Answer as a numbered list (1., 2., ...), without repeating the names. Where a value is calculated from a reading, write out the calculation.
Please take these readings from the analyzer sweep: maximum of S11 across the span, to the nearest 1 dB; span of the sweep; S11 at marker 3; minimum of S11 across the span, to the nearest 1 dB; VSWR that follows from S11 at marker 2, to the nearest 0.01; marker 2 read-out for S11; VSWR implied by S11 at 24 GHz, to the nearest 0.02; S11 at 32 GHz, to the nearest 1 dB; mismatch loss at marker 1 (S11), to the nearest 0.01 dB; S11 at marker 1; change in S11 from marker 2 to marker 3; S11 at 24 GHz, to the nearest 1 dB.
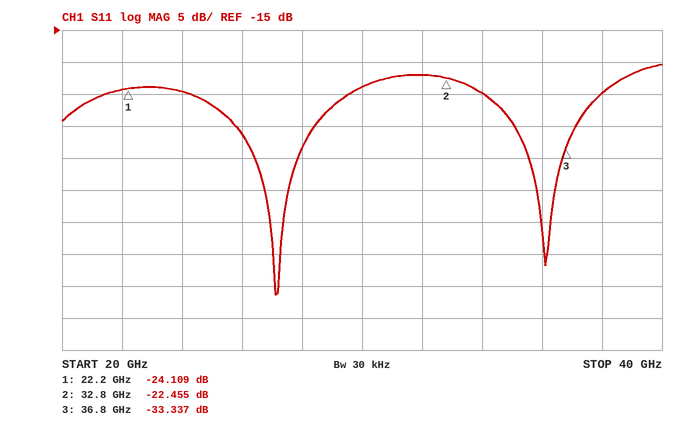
1. -20 dB
2. 20 GHz
3. -33.337 dB
4. -56 dB
5. (1 + 0.0754)/(1 − 0.0754) ≈ 1.16
6. -22.455 dB
7. |Γ| = 10^(-25/20) = 0.0562; VSWR = (1 + 0.0562)/(1 − 0.0562) ≈ 1.12
8. -22 dB
9. −10 log10(1 − 10^(-24.109/10)) ≈ 0.02 dB
10. -24.109 dB
11. -33.337 − (-22.455) = -10.882 dB
12. -25 dB
